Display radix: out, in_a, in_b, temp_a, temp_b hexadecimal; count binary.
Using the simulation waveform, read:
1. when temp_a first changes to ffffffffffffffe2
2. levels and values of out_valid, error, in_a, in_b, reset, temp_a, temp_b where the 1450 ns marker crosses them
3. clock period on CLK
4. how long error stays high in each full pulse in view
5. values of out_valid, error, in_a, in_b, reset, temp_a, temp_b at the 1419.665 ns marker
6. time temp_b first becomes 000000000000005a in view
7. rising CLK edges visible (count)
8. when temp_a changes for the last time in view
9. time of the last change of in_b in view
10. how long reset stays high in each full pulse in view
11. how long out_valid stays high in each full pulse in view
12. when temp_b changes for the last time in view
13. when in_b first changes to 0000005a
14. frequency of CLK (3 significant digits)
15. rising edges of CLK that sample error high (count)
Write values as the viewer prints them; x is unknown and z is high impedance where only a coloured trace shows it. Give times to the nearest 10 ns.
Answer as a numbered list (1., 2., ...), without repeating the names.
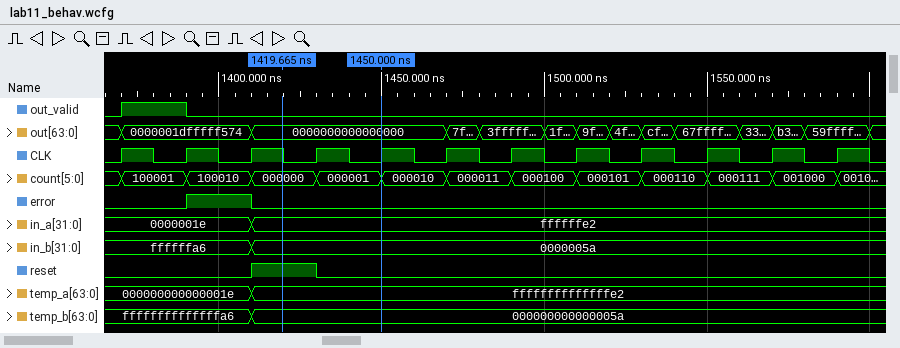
1. 1410 ns
2. out_valid=0, error=0, in_a=ffffffe2, in_b=0000005a, reset=0, temp_a=ffffffffffffffe2, temp_b=000000000000005a
3. 20 ns
4. 20 ns
5. out_valid=0, error=0, in_a=ffffffe2, in_b=0000005a, reset=1, temp_a=ffffffffffffffe2, temp_b=000000000000005a
6. 1410 ns
7. 12
8. 1410 ns
9. 1410 ns
10. 20 ns
11. 20 ns
12. 1410 ns
13. 1410 ns
14. 50.0 MHz
15. 1
